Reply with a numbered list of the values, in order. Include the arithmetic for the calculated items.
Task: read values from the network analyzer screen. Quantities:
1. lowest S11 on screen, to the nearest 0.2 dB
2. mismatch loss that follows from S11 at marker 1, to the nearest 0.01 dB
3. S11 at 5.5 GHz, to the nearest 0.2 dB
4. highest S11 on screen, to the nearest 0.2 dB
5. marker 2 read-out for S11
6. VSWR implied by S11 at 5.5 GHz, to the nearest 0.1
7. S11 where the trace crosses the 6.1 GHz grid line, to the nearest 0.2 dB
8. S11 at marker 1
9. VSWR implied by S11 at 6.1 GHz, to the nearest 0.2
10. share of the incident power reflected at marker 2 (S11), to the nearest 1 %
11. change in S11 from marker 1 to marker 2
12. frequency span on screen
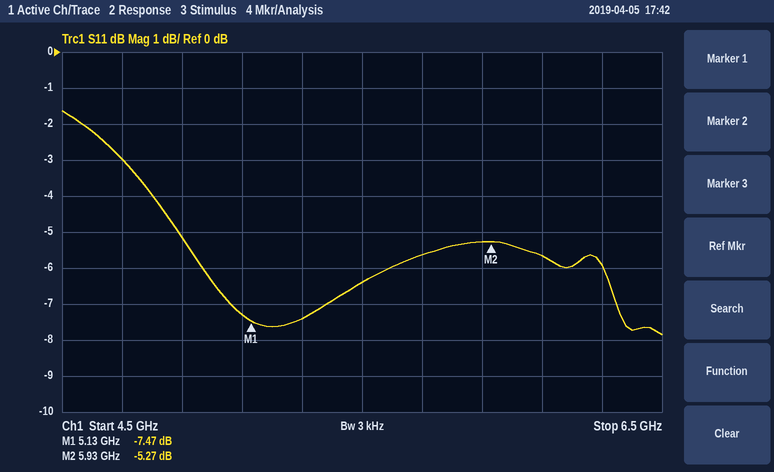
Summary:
1. -7.8 dB
2. −10 log10(1 − 10^(-7.47/10)) ≈ 0.86 dB
3. -6.4 dB
4. -1.6 dB
5. -5.27 dB
6. |Γ| = 10^(-6.4/20) = 0.4786; VSWR = (1 + 0.4786)/(1 − 0.4786) ≈ 2.8
7. -5.6 dB
8. -7.47 dB
9. |Γ| = 10^(-5.6/20) = 0.5248; VSWR = (1 + 0.5248)/(1 − 0.5248) ≈ 3.2
10. 10^(-5.27/10) ≈ 30 %
11. -5.27 − (-7.47) = 2.20 dB
12. 2 GHz
